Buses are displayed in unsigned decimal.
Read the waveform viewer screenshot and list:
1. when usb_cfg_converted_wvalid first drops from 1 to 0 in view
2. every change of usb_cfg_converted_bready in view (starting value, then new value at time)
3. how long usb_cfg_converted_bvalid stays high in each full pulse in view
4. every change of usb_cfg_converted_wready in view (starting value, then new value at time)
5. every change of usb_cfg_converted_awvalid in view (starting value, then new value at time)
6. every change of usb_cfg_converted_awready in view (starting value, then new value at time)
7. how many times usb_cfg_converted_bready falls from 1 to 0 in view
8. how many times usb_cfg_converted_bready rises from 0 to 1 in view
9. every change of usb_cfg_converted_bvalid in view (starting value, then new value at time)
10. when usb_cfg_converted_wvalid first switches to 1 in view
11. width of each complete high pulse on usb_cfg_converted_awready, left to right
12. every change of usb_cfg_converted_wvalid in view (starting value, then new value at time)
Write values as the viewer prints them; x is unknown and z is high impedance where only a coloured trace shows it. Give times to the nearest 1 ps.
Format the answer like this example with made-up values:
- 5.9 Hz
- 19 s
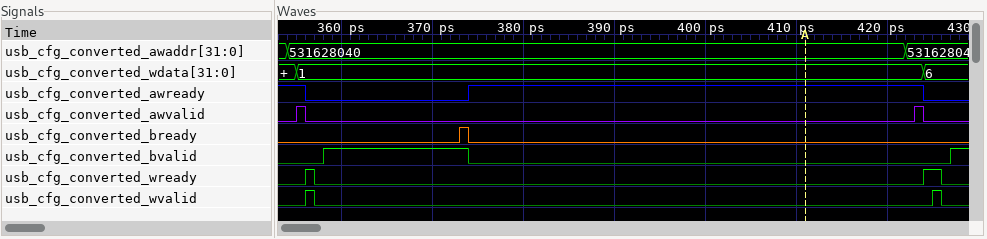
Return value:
- 357 ps
- 0, 1 at 373 ps, 0 at 374 ps
- 16 ps
- 0, 1 at 356 ps, 0 at 357 ps, 1 at 424 ps, 0 at 426 ps
- 0, 1 at 355 ps, 0 at 356 ps, 1 at 423 ps, 0 at 424 ps
- 1, 0 at 356 ps, 1 at 374 ps, 0 at 424 ps
- 1
- 1
- 0, 1 at 358 ps, 0 at 374 ps, 1 at 427 ps
- 356 ps
- 50 ps
- 0, 1 at 356 ps, 0 at 357 ps, 1 at 425 ps, 0 at 426 ps
